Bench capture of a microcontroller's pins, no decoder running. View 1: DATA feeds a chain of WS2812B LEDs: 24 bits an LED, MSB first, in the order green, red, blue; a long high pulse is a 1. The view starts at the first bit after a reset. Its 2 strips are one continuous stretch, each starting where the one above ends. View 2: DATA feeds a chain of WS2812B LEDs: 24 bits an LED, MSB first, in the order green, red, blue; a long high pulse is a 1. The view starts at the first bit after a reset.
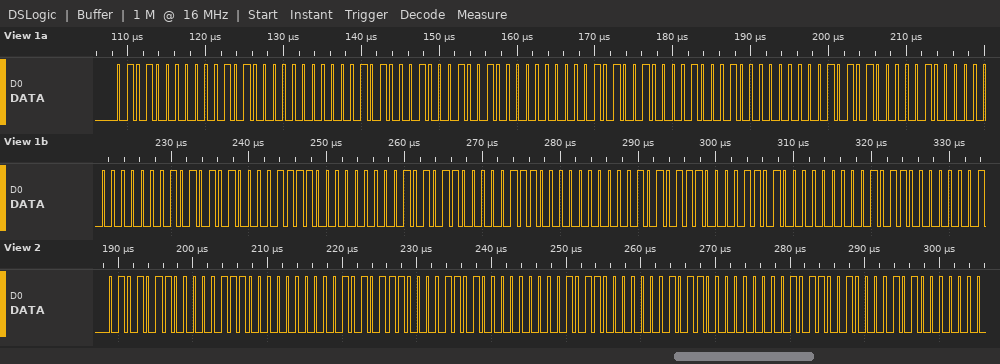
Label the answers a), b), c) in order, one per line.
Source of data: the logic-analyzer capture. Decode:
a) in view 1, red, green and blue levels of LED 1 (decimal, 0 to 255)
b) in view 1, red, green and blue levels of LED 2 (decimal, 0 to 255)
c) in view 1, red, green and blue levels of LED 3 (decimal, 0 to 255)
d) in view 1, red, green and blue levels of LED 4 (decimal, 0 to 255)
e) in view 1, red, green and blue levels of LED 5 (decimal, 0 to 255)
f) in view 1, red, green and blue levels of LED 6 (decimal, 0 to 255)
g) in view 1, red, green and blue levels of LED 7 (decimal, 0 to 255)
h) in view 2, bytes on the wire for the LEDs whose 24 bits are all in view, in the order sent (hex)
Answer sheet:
a) 20, 80, 0
b) 18, 81, 0
c) 17, 82, 0
d) 16, 84, 0
e) 15, 85, 0
f) 14, 86, 0
g) 13, 87, 0
h) 56 0E 00 57 0D 00 58 0B 00
